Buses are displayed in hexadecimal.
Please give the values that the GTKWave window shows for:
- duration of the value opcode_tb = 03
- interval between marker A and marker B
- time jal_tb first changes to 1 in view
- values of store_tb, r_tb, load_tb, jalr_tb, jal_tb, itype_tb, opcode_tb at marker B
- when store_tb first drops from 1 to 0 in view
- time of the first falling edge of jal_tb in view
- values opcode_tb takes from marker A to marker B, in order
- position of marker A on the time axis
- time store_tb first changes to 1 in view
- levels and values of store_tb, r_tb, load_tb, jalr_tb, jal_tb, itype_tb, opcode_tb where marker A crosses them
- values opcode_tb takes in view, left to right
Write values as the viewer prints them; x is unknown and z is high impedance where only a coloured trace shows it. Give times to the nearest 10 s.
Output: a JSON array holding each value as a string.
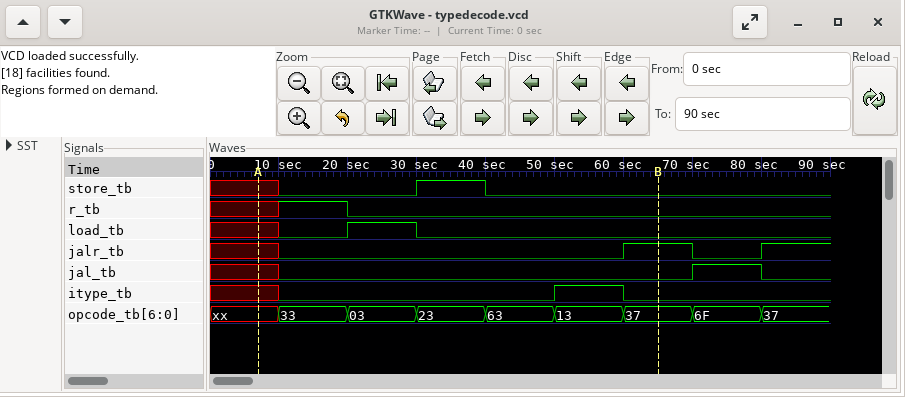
["10 s", "60 s", "70 s", "store_tb=0, r_tb=0, load_tb=0, jalr_tb=1, jal_tb=0, itype_tb=0, opcode_tb=37", "40 s", "80 s", "xx, 33, 03, 23, 63, 13, 37", "10 s", "30 s", "store_tb=x, r_tb=x, load_tb=x, jalr_tb=x, jal_tb=x, itype_tb=x, opcode_tb=xx", "xx, 33, 03, 23, 63, 13, 37, 6F, 37"]
